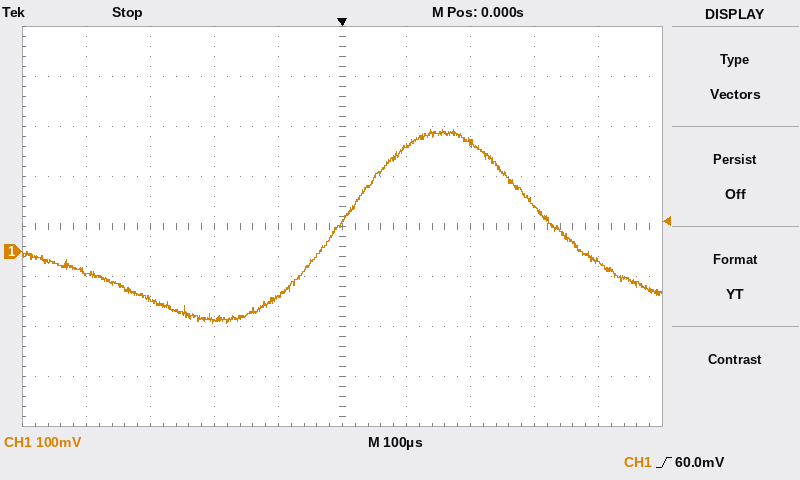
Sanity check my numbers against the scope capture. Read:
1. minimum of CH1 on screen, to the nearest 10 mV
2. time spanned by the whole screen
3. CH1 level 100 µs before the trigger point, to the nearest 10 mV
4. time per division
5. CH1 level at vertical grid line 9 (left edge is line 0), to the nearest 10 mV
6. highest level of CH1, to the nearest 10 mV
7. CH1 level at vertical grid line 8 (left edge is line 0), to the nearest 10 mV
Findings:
-140 mV
1 ms
-90 mV
100 µs
-20 mV
240 mV
90 mV
